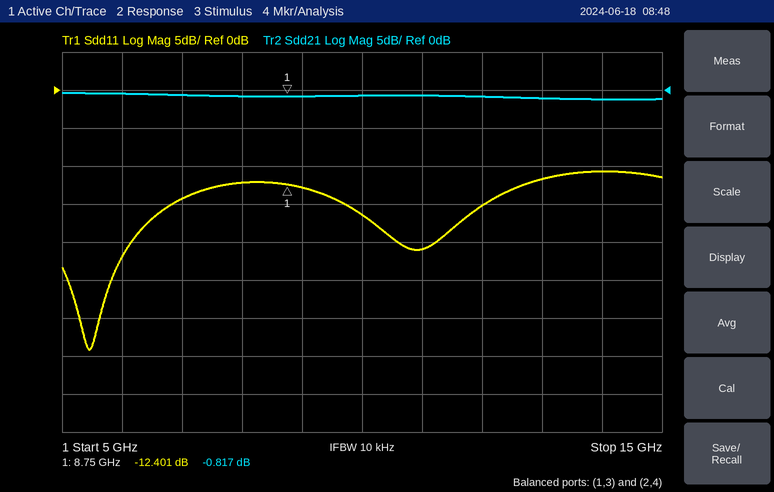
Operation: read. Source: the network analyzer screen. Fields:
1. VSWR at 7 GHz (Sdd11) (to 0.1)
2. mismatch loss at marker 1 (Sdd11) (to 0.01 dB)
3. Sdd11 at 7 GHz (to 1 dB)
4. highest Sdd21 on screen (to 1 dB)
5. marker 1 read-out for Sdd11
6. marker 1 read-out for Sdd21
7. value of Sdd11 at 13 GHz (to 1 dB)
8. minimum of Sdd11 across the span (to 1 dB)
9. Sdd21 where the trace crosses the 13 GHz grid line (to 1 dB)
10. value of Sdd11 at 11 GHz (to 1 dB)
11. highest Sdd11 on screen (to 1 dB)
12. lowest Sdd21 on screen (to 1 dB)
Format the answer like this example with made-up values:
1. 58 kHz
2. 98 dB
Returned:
1. 1.5
2. 0.26 dB
3. -14 dB
4. 0 dB
5. -12.401 dB
6. -0.817 dB
7. -12 dB
8. -34 dB
9. -1 dB
10. -21 dB
11. -11 dB
12. -1 dB
